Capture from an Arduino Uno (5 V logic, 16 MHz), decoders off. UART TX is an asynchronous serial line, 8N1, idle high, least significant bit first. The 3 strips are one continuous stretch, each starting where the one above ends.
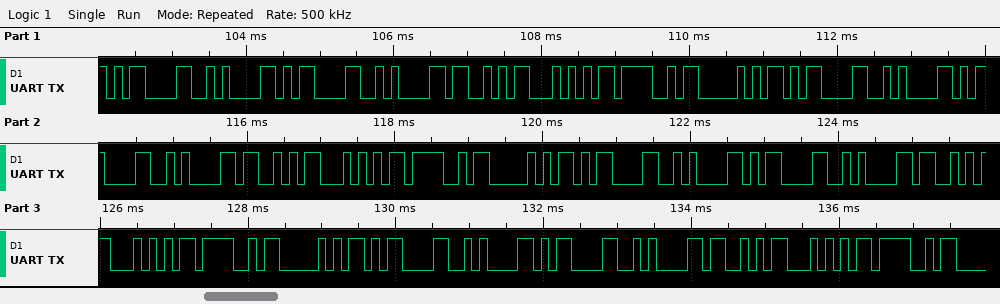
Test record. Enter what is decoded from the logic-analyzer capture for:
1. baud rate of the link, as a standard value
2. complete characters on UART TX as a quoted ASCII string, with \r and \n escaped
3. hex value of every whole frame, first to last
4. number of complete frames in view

9600 baud
"\r\n\r\nSTOP\r\n\r\nSTOP\r\n\r\nSTOP\r\n\r\nSTO"
0D 0A 0D 0A 53 54 4F 50 0D 0A 0D 0A 53 54 4F 50 0D 0A 0D 0A 53 54 4F 50 0D 0A 0D 0A 53 54 4F
31
